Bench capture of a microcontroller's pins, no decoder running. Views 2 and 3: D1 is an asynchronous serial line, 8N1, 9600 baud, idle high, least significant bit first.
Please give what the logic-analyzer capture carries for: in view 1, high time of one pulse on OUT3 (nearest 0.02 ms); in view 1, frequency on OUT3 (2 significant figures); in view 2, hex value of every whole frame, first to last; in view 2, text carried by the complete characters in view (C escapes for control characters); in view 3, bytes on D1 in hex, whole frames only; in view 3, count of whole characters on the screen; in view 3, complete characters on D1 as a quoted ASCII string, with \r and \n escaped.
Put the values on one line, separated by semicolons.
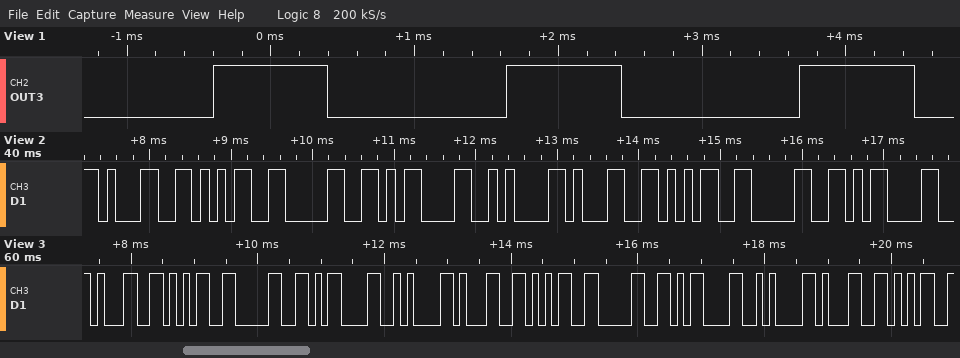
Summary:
0.80 ms; 490 Hz; 31 35 30 0D 0A 31 35 30 0D; "150\r\n150\r"; 0x31 0x35 0x30 0x0D 0x0A 0x31 0x35 0x30 0x0D 0x0A 0x31 0x35; 12; "150\r\n150\r\n15"
